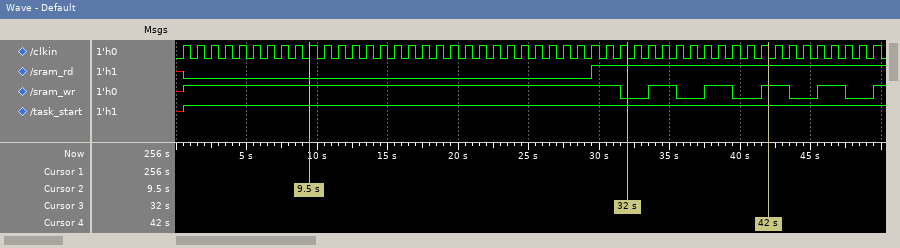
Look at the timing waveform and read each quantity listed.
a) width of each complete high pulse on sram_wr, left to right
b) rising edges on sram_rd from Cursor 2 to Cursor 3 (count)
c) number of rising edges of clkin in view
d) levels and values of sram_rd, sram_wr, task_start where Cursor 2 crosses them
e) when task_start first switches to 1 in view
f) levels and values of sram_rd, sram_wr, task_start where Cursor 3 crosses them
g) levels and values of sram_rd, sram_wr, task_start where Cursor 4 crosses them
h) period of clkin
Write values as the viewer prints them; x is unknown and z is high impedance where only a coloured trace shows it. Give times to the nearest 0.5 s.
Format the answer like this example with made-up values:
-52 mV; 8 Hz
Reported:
2 s, 2 s, 2 s, 2 s; 1; 50; sram_rd=0, sram_wr=1, task_start=1; 0.5 s; sram_rd=1, sram_wr=0, task_start=1; sram_rd=1, sram_wr=1, task_start=1; 1 s
